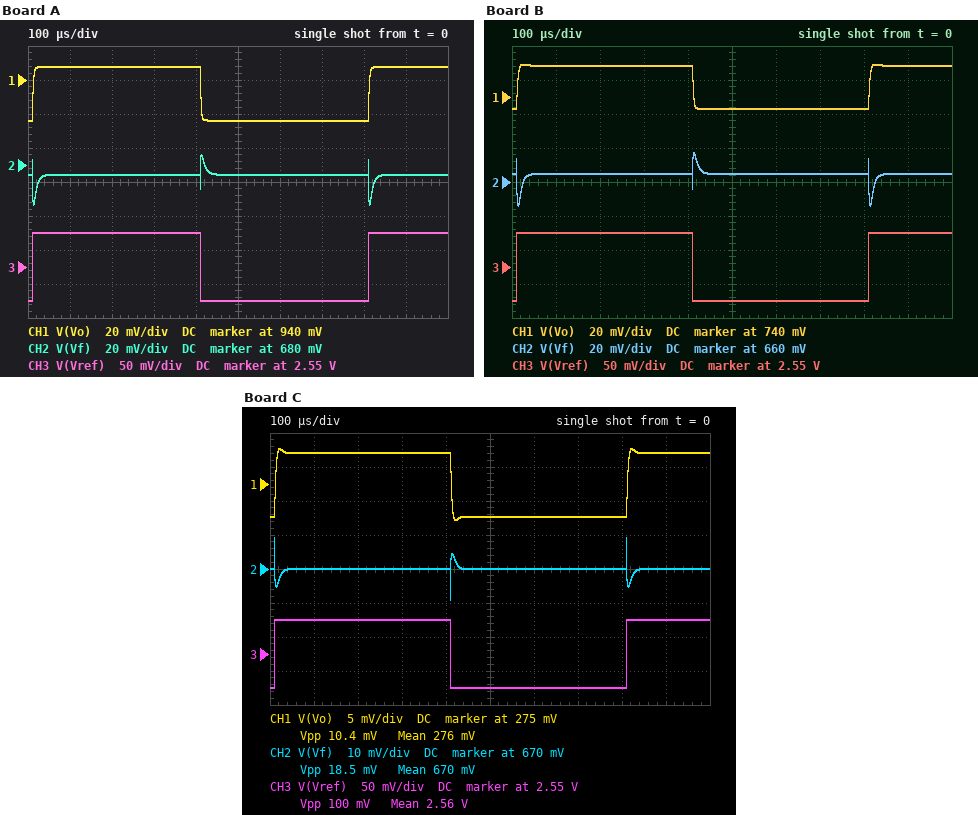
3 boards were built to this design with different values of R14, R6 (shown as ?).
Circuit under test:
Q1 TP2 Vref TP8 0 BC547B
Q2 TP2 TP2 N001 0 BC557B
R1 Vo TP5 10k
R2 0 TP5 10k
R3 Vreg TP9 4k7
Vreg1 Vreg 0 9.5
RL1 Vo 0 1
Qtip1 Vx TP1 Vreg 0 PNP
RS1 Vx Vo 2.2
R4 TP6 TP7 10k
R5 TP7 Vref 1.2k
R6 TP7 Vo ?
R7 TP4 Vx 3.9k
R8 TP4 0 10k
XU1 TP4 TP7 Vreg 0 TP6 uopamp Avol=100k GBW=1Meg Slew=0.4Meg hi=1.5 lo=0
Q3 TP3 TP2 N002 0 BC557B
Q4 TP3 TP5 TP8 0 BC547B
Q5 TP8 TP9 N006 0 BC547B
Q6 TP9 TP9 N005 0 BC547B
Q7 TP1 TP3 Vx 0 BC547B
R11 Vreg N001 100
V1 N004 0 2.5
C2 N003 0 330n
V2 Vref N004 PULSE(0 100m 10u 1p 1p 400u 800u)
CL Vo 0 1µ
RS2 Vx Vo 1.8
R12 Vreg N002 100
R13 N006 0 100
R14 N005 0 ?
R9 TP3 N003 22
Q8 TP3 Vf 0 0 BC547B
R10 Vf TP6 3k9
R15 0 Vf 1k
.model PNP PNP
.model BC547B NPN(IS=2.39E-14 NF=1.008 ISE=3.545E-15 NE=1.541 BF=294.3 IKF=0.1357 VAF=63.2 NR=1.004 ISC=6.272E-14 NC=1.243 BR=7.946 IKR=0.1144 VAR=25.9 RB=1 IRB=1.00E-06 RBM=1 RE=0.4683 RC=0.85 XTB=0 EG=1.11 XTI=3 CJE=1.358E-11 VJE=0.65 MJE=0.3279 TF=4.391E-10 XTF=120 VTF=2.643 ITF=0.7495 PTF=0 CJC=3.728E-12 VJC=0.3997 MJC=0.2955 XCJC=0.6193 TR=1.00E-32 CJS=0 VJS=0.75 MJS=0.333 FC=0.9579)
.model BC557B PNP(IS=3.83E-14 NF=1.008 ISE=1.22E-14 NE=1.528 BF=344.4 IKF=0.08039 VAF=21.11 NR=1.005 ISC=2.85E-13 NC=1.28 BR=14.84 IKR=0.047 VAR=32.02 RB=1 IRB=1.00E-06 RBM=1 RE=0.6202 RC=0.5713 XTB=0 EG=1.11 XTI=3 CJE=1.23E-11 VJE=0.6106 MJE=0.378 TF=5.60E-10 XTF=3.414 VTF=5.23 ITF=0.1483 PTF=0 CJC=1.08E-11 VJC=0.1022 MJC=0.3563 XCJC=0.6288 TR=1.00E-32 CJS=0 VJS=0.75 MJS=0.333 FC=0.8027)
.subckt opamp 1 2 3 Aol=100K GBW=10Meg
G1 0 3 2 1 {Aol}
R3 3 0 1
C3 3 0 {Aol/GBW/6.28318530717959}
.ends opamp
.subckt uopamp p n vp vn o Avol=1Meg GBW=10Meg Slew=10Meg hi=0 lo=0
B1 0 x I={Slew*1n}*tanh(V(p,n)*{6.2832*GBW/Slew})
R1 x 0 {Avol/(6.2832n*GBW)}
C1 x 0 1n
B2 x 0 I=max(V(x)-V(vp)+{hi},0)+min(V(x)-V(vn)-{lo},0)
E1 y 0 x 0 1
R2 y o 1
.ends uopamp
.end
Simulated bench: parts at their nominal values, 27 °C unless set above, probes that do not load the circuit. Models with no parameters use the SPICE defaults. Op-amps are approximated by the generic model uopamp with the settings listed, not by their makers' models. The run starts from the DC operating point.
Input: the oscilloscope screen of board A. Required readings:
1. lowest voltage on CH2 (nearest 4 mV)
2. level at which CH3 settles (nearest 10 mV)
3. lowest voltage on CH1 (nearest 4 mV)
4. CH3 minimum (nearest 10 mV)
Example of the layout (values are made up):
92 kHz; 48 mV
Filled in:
656 mV; 2.60 V; 916 mV; 2.50 V
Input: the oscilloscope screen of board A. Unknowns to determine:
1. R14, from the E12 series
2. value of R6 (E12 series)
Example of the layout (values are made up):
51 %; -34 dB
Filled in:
220 Ω; 330 Ω
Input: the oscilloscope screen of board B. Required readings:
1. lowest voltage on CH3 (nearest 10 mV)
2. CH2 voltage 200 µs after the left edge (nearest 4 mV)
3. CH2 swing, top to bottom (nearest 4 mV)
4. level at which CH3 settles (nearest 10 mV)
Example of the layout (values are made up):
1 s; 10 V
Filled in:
2.50 V; 664 mV; 32 mV; 2.60 V
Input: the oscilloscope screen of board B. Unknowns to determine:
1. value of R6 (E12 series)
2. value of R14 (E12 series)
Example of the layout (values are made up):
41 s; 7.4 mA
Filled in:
220 Ω; 150 Ω
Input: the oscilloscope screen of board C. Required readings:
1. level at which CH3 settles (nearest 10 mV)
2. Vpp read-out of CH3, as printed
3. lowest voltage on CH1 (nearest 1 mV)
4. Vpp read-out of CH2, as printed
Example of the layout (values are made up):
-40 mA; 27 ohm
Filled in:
2.60 V; 100 mV; 270 mV; 18.5 mV
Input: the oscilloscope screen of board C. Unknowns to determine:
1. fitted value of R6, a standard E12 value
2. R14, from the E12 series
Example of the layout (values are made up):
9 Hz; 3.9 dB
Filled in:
56 Ω; 180 Ω
